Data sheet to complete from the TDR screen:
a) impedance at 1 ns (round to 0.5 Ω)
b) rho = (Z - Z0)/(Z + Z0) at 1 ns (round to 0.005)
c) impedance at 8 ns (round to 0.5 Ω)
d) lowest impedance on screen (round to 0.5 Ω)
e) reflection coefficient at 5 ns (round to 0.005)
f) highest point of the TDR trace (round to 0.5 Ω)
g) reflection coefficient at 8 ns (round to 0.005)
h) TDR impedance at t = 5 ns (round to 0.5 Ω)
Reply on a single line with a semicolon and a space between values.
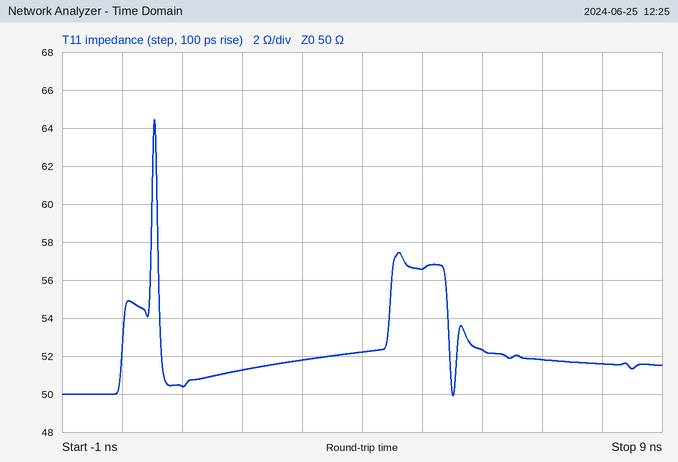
50.5 Ω; +0.005; 51.5 Ω; 50.0 Ω; +0.060; 64.5 Ω; +0.015; 56.5 Ω
